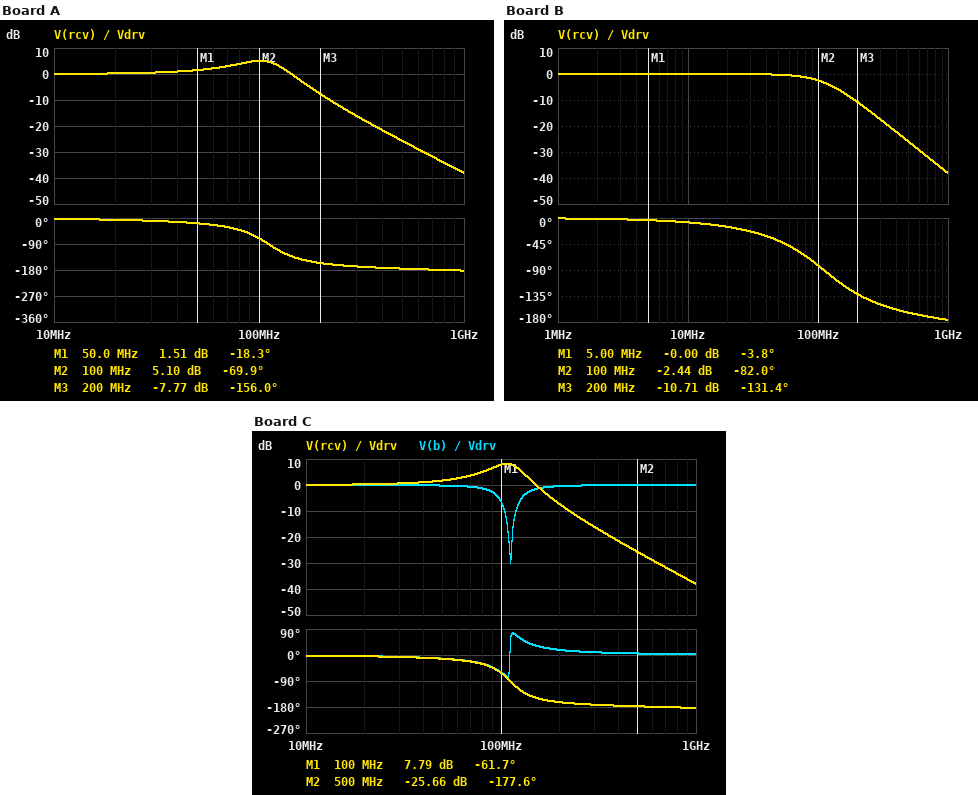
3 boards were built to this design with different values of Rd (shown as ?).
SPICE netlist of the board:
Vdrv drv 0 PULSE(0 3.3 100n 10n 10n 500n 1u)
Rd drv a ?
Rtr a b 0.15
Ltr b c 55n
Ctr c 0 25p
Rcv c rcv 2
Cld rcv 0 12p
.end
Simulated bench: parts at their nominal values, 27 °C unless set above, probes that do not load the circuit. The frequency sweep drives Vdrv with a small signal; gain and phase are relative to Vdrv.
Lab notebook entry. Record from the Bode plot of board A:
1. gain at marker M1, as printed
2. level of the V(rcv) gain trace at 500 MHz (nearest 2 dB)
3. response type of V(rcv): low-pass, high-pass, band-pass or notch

1.51 dB
-26 dB
low-pass
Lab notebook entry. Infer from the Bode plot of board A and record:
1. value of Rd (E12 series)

22 Ω
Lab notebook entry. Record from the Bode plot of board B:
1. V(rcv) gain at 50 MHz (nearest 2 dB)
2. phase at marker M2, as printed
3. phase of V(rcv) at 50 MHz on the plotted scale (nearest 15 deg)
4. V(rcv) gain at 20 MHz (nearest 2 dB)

0 dB
-82.0 deg
-45 deg
0 dB
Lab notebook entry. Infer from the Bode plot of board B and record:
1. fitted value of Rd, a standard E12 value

56 Ω
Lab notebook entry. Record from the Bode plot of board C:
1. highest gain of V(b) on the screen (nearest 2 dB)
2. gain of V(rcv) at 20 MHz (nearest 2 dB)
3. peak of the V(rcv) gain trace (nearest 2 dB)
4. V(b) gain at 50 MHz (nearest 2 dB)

0 dB
0 dB
8 dB
0 dB
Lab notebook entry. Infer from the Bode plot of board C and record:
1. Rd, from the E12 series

15 Ω
